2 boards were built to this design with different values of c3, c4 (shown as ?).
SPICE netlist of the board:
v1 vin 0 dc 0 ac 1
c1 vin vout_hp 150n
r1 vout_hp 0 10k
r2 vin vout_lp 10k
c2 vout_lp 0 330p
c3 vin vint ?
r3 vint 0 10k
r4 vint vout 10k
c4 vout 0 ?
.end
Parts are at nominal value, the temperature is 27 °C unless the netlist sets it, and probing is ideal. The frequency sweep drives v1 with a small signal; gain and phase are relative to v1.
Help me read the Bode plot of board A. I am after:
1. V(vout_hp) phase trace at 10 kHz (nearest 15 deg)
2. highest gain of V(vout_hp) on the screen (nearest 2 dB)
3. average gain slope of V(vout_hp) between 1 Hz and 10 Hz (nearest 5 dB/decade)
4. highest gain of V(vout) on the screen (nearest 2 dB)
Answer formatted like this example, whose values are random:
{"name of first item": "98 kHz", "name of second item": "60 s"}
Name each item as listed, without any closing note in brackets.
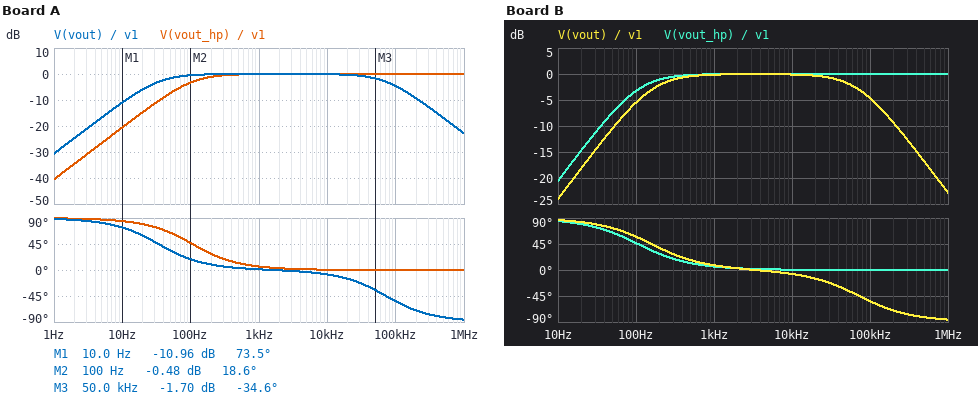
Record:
{"V(vout_hp) phase trace at 10 kHz": "0 deg", "highest gain of V(vout_hp) on the screen": "0 dB", "average gain slope of V(vout_hp) between 1 Hz and 10 Hz": "20 dB/decade", "highest gain of V(vout) on the screen": "0 dB"}
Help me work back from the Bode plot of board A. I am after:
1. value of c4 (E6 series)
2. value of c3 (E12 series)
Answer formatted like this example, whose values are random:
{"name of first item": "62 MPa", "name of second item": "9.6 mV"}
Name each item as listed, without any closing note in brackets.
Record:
{"value of c4": "220 pF", "value of c3": "470 nF"}
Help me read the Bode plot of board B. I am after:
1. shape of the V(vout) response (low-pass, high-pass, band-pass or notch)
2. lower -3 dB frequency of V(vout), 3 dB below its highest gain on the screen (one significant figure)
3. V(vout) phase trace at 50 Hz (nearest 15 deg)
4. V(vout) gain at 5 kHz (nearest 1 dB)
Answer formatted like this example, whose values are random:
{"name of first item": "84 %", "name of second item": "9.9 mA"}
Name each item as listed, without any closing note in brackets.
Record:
{"shape of the V(vout) response": "band-pass", "lower -3 dB frequency of V(vout), 3 dB below its highest gain on the screen": "200 Hz", "V(vout) phase trace at 50 Hz": "75 deg", "V(vout) gain at 5 kHz": "0 dB"}
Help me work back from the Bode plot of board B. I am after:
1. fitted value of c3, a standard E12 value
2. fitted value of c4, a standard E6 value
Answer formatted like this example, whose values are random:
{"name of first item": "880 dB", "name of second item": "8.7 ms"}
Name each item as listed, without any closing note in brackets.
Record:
{"fitted value of c3, a standard E12 value": "100 nF", "fitted value of c4, a standard E6 value": "220 pF"}
